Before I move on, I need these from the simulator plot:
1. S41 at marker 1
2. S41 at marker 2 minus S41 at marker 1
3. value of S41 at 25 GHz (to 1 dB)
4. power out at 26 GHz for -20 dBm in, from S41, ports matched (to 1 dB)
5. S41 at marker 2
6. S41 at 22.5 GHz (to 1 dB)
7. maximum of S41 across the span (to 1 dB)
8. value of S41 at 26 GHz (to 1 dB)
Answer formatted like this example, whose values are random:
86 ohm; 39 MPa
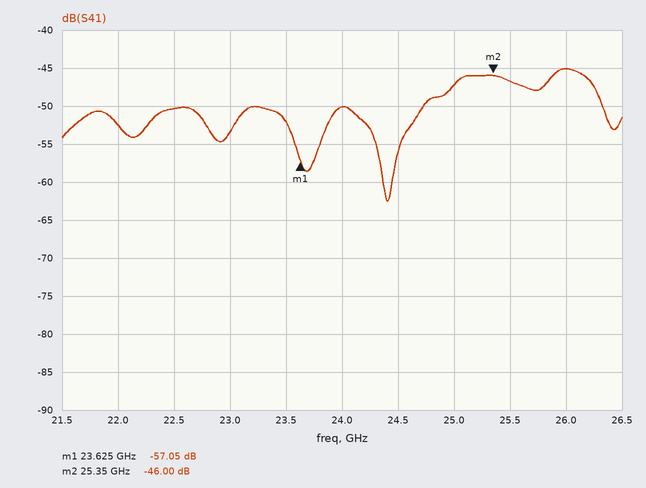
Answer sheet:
-57.05 dB; 11.05 dB; -47 dB; -65 dBm; -46.00 dB; -50 dB; -45 dB; -45 dB
